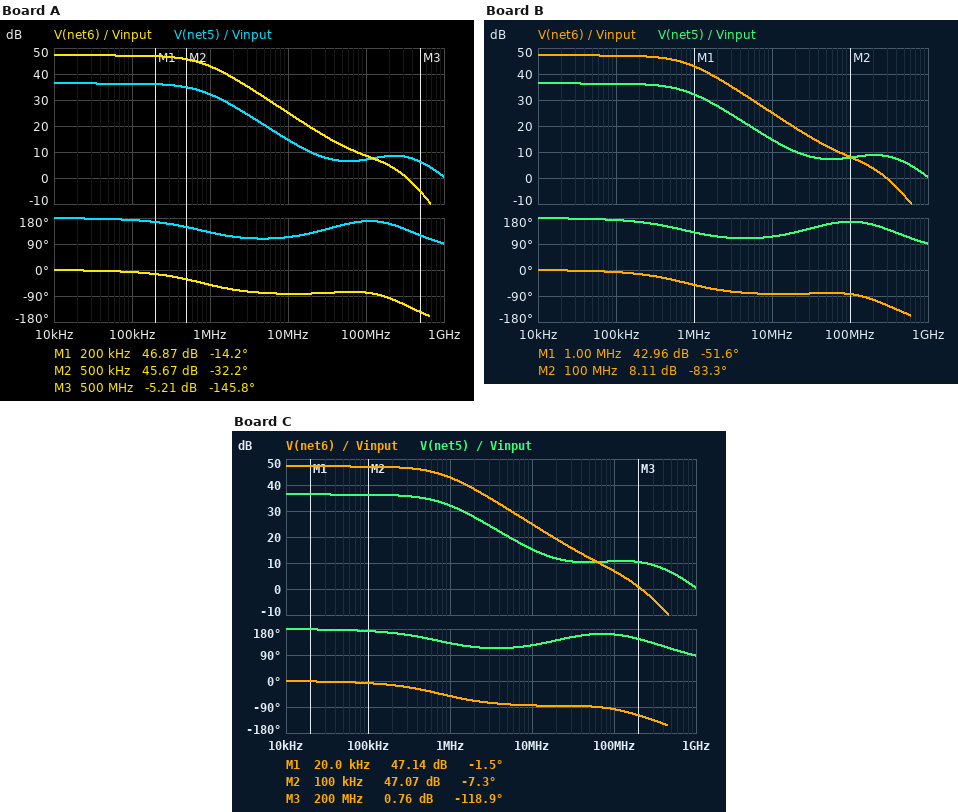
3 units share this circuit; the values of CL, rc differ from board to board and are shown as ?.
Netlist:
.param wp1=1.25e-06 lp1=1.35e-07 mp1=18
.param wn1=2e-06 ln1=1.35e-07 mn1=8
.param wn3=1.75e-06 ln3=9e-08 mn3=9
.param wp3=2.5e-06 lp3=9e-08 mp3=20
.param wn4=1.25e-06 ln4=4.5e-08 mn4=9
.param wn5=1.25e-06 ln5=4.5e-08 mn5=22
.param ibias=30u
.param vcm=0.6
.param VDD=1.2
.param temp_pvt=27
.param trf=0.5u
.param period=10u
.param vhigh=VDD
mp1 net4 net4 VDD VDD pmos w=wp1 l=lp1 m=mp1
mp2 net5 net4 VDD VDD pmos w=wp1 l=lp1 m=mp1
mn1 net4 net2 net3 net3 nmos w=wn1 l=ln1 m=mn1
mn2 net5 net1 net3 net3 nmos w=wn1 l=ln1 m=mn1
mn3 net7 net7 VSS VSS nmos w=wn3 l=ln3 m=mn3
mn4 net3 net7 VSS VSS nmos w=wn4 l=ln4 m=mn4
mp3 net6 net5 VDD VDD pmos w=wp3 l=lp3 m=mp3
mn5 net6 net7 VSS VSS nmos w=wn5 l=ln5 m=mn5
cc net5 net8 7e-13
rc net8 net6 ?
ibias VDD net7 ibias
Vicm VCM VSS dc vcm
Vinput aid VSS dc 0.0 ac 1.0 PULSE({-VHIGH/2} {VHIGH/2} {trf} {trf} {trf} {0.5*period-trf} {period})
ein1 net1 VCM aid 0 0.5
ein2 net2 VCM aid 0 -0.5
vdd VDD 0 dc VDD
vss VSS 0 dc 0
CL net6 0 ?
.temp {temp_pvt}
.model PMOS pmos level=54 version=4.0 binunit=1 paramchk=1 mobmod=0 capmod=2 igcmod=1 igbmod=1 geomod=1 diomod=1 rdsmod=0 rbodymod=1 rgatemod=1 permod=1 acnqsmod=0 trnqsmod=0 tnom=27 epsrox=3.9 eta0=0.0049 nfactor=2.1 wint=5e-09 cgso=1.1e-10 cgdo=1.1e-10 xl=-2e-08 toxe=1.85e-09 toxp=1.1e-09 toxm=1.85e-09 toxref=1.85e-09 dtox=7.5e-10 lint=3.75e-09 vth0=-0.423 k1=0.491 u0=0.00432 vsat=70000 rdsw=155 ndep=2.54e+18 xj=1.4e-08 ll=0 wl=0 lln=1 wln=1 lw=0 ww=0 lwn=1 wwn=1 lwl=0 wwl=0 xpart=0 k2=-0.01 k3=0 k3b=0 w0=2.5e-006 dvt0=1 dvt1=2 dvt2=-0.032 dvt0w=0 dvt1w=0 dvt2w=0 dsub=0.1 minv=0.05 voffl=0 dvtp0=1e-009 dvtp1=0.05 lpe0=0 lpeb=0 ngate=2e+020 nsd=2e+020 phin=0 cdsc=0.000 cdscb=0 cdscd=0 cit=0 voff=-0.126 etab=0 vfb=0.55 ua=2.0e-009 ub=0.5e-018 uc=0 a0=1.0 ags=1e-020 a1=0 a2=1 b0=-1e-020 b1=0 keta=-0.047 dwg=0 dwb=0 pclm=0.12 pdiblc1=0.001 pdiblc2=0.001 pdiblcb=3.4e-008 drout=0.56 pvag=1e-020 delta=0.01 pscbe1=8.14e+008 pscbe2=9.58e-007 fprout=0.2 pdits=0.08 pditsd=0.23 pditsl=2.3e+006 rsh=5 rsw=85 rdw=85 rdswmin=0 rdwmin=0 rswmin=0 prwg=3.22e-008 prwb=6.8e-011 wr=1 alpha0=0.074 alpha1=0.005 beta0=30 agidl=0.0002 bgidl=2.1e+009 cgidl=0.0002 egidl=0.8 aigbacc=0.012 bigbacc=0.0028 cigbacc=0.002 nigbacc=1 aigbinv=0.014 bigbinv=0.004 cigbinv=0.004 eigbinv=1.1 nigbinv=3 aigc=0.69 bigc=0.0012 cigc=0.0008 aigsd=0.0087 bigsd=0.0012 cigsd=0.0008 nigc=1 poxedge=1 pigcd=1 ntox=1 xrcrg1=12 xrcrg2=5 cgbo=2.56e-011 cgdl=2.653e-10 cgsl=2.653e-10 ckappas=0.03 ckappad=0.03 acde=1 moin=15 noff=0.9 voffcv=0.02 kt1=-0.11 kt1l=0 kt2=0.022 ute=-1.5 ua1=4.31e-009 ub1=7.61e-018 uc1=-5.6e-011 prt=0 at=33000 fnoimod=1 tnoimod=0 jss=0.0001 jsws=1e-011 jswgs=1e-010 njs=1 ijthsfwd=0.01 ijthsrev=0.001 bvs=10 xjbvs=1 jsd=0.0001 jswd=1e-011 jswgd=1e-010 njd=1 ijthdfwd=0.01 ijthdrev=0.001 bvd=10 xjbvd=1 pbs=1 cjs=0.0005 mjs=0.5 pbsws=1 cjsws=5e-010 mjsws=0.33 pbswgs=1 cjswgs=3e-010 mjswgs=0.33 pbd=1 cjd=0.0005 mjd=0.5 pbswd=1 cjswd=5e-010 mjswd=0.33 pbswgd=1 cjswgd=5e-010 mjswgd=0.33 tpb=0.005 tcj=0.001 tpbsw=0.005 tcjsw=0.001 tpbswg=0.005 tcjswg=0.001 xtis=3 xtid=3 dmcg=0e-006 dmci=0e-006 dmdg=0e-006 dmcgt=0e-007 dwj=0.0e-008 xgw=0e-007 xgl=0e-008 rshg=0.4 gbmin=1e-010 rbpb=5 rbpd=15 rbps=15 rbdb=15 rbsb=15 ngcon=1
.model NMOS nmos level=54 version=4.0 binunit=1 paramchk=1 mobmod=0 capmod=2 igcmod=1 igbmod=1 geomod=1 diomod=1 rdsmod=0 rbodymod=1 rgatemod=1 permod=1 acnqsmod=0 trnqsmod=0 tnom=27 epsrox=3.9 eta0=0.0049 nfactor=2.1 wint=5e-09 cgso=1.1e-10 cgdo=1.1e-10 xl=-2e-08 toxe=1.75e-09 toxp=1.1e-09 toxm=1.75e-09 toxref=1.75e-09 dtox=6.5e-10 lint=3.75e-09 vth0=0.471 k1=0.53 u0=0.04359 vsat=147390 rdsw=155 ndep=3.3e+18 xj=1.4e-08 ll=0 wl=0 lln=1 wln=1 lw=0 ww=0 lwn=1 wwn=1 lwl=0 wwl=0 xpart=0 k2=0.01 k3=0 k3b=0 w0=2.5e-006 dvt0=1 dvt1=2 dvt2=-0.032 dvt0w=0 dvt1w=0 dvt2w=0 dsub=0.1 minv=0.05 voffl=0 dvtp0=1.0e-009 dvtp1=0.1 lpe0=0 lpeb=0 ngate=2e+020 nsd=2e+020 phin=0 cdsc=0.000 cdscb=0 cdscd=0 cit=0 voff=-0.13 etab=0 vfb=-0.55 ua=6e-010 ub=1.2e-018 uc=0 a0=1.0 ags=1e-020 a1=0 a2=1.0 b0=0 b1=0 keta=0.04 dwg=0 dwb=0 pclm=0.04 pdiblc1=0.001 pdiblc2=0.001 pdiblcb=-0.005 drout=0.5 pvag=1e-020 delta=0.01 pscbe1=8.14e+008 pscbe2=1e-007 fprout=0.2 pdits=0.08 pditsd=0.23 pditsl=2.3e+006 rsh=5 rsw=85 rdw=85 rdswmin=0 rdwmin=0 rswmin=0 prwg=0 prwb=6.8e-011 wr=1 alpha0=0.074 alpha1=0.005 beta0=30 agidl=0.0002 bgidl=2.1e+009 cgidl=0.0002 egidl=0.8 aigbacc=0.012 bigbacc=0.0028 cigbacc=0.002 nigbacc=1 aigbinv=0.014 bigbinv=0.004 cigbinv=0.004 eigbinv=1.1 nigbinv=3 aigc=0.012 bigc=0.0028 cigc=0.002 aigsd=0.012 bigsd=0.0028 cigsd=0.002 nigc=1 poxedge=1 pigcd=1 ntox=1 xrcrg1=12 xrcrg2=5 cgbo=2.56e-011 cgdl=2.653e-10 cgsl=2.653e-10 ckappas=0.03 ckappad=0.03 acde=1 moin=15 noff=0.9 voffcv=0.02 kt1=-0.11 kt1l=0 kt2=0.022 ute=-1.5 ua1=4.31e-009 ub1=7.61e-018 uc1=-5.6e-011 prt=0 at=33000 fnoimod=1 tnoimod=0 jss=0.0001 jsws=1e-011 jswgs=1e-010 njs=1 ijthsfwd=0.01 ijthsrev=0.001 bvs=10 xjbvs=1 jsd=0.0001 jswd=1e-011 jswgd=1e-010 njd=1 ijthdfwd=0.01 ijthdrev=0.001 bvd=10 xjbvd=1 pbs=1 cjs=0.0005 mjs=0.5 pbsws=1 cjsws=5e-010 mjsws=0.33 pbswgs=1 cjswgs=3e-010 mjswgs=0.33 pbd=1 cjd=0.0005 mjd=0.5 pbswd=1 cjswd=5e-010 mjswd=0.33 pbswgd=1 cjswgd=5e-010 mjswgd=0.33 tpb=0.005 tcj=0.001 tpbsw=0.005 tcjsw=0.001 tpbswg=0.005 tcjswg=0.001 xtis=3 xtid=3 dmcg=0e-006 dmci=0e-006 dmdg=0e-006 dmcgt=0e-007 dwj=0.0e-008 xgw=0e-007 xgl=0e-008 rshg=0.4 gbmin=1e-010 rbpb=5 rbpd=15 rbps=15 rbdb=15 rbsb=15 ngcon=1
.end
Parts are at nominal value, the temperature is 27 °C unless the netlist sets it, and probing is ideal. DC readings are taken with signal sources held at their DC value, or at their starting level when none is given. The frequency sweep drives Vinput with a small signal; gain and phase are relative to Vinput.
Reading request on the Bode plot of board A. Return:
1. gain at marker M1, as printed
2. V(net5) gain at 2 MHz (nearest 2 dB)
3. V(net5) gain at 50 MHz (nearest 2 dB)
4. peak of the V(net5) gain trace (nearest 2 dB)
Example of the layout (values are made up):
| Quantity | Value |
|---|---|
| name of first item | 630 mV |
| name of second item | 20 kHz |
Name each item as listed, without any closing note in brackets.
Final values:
| Quantity | Value |
|---|---|
| gain at marker M1, as printed | 46.87 dB |
| V(net5) gain at 2 MHz | 28 dB |
| V(net5) gain at 50 MHz | 6 dB |
| peak of the V(net5) gain trace | 36 dB |
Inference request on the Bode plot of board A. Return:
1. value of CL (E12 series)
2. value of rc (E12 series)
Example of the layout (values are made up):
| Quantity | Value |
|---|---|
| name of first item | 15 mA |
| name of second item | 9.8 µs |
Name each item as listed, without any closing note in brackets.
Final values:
| Quantity | Value |
|---|---|
| value of CL | 3.9 pF |
| value of rc | 3.3 kΩ |
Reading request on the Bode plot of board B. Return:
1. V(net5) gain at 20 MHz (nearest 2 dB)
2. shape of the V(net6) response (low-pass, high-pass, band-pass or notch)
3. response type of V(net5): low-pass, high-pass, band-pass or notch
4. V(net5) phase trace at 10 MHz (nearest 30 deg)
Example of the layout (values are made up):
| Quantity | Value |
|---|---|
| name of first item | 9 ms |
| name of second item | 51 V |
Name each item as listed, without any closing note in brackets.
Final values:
| Quantity | Value |
|---|---|
| V(net5) gain at 20 MHz | 10 dB |
| shape of the V(net6) response | low-pass |
| response type of V(net5): low-pass, high-pass, band-pass or notch | low-pass |
| V(net5) phase trace at 10 MHz | 120 deg |
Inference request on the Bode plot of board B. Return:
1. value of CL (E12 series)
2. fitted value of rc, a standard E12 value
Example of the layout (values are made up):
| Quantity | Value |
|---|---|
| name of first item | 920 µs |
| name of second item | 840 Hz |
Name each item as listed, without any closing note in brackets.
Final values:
| Quantity | Value |
|---|---|
| value of CL | 4.7 pF |
| fitted value of rc, a standard E12 value | 3.3 kΩ |
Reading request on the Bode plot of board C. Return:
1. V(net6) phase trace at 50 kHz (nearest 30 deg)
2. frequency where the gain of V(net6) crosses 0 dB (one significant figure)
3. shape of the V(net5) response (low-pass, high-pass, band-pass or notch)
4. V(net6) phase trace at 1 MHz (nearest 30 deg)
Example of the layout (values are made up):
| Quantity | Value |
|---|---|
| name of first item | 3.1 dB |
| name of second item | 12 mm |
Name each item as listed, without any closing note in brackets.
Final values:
| Quantity | Value |
|---|---|
| V(net6) phase trace at 50 kHz | 0 deg |
| frequency where the gain of V(net6) crosses 0 dB | 200 MHz |
| shape of the V(net5) response | low-pass |
| V(net6) phase trace at 1 MHz | -60 deg |
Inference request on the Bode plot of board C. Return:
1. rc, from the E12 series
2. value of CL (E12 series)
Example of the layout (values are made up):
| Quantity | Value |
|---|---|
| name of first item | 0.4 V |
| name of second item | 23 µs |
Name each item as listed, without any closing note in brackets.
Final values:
| Quantity | Value |
|---|---|
| rc, from the E12 series | 3.9 kΩ |
| value of CL | 8.2 pF |
